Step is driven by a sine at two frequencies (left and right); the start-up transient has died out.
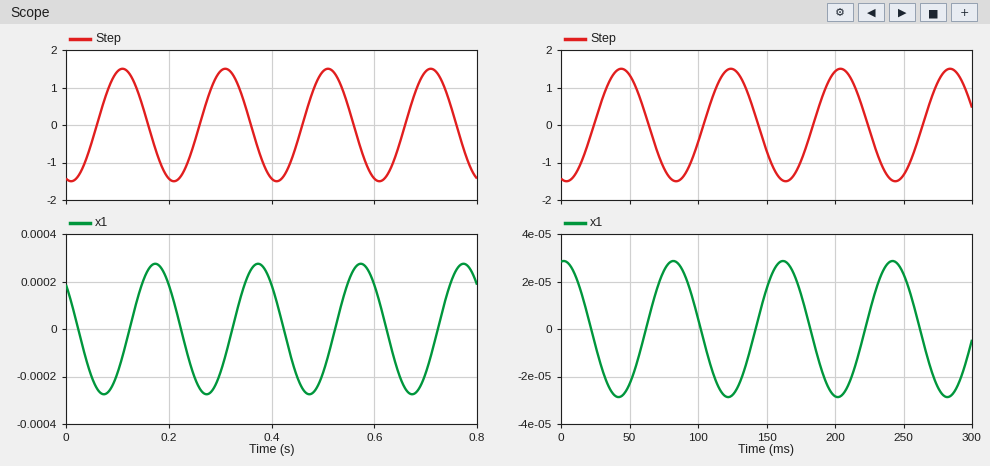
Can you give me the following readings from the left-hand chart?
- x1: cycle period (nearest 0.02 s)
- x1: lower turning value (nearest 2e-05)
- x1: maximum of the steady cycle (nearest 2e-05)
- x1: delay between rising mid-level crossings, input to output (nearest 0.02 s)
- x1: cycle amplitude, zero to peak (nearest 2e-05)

0.20 s
-0.00028
0.00028
0.06 s
0.00028
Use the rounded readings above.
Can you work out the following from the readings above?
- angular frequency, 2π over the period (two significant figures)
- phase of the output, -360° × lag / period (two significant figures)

31 rad/s
-110°
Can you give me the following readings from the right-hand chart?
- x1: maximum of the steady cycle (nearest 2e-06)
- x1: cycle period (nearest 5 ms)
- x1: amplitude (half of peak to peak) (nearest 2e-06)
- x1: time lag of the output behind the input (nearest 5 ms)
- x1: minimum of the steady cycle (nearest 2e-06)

0.000028
80 ms
0.000028
40 ms
-0.000028
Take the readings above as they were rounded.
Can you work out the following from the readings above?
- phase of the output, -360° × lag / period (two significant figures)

-180°
